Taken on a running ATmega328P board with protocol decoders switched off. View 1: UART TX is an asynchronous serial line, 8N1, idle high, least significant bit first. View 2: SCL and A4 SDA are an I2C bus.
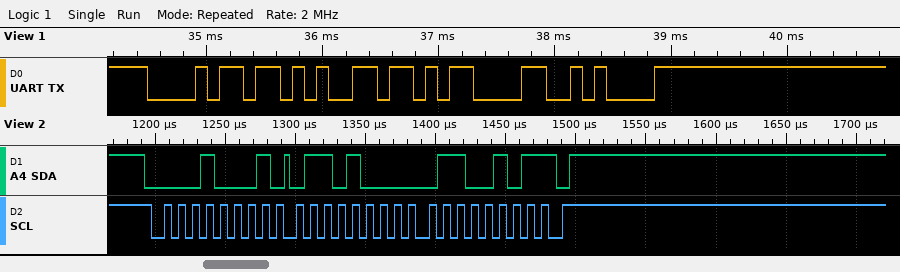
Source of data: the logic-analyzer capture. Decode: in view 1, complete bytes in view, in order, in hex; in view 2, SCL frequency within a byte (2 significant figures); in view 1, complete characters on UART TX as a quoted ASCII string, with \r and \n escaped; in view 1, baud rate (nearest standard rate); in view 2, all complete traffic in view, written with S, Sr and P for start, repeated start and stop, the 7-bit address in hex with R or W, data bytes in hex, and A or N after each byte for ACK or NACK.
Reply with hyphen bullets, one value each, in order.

- 0x68 0x65 0x0D 0x0A
- 100 kHz
- "he\r\n"
- 9600 baud
- S 08R A 68 A 65 N P
